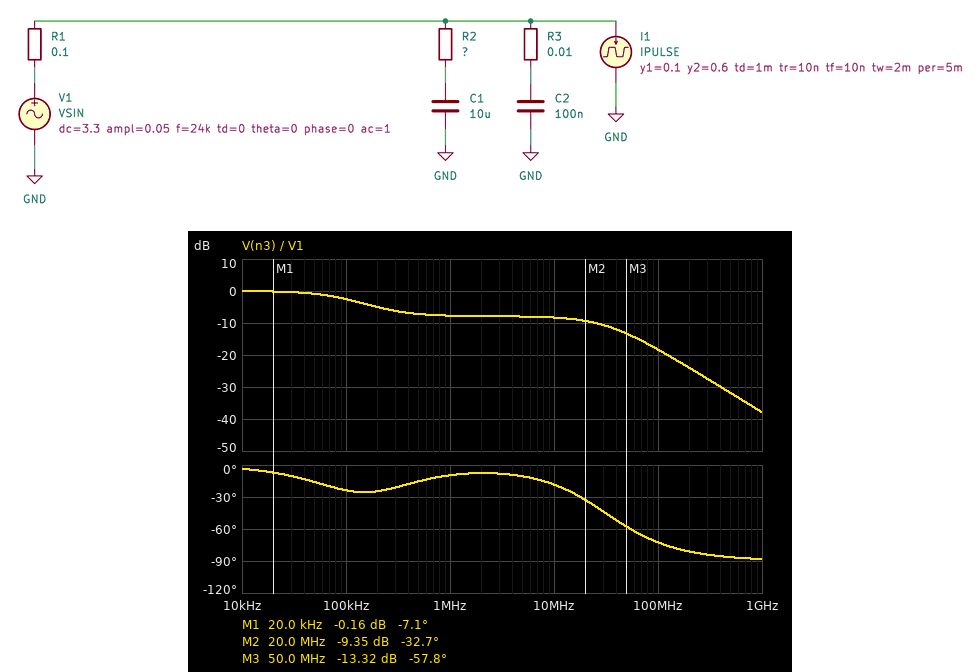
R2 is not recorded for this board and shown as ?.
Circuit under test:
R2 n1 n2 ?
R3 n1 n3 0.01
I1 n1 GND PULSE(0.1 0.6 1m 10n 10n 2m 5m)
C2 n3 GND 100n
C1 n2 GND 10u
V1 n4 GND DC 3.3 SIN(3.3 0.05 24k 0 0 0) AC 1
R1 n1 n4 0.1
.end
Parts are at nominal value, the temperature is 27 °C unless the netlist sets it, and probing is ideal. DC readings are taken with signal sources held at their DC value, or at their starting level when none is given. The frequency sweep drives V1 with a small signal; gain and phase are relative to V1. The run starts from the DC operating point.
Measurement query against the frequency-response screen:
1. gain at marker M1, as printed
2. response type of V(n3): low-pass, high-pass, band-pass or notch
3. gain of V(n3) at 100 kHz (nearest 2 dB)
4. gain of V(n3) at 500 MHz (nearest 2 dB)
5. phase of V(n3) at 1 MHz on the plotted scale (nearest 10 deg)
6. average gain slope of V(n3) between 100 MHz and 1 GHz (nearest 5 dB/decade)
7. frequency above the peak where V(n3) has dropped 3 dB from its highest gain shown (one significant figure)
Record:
-0.16 dB
low-pass
-2 dB
-32 dB
-10 deg
-20 dB/decade
100 kHz
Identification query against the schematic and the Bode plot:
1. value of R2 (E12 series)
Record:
0.068 Ω
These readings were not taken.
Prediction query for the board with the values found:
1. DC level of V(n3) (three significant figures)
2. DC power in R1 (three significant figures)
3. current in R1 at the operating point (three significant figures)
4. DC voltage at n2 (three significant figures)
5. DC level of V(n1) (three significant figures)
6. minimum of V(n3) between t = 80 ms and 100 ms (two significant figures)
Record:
3.29 V
1.00 mW
100 mA
3.29 V
3.29 V
3.2 V
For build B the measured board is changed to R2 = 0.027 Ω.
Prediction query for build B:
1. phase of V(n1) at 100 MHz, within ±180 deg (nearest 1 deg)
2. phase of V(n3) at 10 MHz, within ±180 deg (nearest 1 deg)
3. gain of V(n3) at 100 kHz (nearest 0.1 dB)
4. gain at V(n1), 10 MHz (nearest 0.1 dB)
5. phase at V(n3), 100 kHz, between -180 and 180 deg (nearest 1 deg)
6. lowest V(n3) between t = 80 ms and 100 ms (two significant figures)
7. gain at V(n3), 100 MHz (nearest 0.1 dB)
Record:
-31 deg
-14 deg
-2.0 dB
-13.6 dB
-29 deg
3.2 V
-20.3 dB
